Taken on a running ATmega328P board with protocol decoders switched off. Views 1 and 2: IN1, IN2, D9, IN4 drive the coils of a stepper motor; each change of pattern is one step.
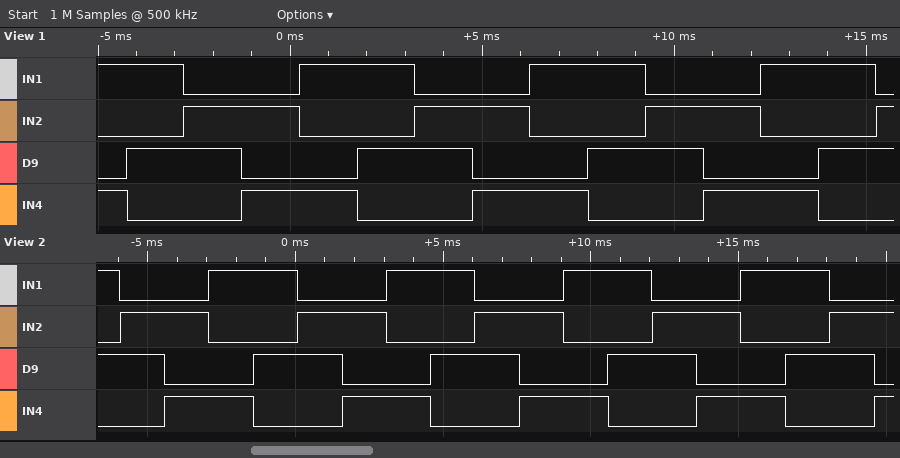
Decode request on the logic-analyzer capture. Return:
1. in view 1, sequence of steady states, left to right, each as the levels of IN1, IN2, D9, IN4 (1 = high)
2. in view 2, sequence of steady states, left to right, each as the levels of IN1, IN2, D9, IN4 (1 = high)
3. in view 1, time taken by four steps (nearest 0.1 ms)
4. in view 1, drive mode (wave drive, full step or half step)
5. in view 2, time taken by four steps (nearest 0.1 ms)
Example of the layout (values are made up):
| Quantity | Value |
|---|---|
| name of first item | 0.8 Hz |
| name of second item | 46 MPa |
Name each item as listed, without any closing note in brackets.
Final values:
| Quantity | Value |
|---|---|
| in view 1, sequence of steady states, left to right, each as the levels of IN1, IN2, D9, IN4 | 1001 1010 0110 0101 1001 1010 0110 0101 1001 1010 0110 0101 1001 1010 0110 |
| in view 2, sequence of steady states, left to right, each as the levels of IN1, IN2, D9, IN4 | 1010 0110 0101 1001 1010 0110 0101 1001 1010 0110 0101 1001 1010 0110 0101 1001 1010 0110 0101 |
| in view 1, time taken by four steps | 6.0 ms |
| in view 1, drive mode | full step |
| in view 2, time taken by four steps | 6.0 ms |
